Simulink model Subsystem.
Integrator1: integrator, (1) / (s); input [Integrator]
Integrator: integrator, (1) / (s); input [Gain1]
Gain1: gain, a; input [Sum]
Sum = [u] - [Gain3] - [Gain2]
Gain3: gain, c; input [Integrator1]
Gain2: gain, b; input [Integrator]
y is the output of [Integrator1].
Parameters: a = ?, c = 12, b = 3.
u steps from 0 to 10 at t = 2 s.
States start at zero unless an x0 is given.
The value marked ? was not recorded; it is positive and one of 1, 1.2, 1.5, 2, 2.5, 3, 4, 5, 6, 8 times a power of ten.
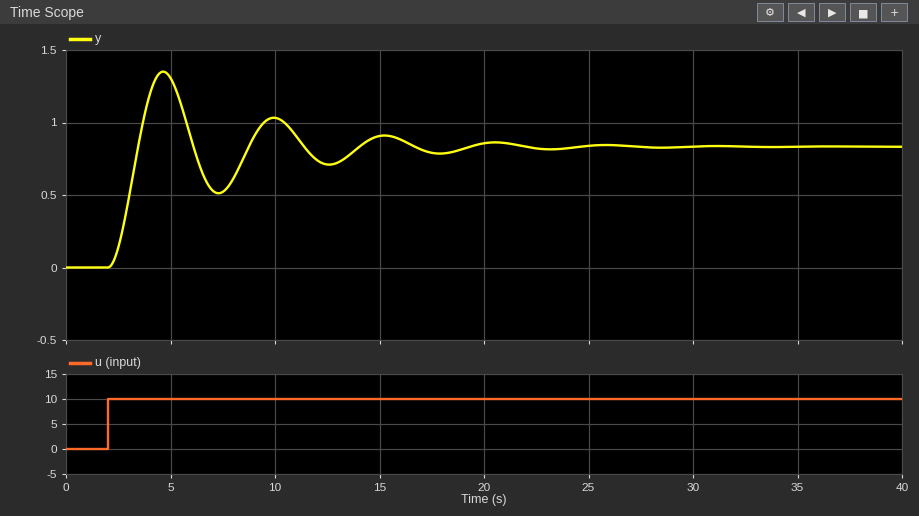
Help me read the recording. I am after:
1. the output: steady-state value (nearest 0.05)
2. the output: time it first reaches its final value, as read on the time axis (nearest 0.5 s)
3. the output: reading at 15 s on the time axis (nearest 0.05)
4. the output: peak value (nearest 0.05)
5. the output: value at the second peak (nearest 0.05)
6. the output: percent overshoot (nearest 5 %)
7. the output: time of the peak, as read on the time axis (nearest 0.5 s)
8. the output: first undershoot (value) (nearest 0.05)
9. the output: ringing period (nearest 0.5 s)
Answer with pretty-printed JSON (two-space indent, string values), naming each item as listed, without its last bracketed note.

{
  "the output: steady-state value": "0.85",
  "the output: time it first reaches its final value, as read on the time axis": "3.5 s",
  "the output: reading at 15 s on the time axis": "0.90",
  "the output: peak value": "1.35",
  "the output: value at the second peak": "1.05",
  "the output: percent overshoot": "60 %",
  "the output: time of the peak, as read on the time axis": "4.5 s",
  "the output: first undershoot (value)": "0.50",
  "the output: ringing period": "5.5 s"
}
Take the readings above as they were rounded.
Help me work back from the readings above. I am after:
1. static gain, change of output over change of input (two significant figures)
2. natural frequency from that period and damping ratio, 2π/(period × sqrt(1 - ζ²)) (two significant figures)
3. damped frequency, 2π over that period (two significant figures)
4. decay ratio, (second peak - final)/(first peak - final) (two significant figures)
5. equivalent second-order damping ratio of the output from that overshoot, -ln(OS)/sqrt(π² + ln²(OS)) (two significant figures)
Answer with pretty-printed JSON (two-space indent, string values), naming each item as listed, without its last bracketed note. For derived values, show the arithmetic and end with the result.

{
  "static gain, change of output over change of input": "(0.85 - 0) / (10 - 0) = 0.085",
  "natural frequency from that period and damping ratio, 2π/(period × sqrt(1 - ζ²))": "2π / (5.5 × sqrt(1 - 0.16²)) = 1.2 rad/s",
  "damped frequency, 2π over that period": "2π / 5.5 = 1.1 rad/s",
  "decay ratio, (second peak - final)/(first peak - final)": "(1.05 - 0.85) / (1.35 - 0.85) = 0.40",
  "equivalent second-order damping ratio of the output from that overshoot, -ln(OS)/sqrt(π² + ln²(OS))": "ln(0.6) = -0.511; 0.511 / sqrt(9.870 + 0.261) = 0.16"
}
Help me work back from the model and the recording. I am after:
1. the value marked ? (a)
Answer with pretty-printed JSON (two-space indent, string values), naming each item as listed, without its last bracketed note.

{
  "the value marked ?": "0.12"
}
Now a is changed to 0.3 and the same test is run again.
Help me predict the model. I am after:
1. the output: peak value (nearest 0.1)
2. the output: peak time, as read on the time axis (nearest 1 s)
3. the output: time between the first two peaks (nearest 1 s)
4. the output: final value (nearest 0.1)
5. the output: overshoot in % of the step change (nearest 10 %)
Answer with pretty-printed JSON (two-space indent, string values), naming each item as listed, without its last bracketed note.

{
  "the output: peak value": "1.2",
  "the output: peak time, as read on the time axis": "4 s",
  "the output: time between the first two peaks": "3 s",
  "the output: final value": "0.8",
  "the output: overshoot in % of the step change": "50 %"
}
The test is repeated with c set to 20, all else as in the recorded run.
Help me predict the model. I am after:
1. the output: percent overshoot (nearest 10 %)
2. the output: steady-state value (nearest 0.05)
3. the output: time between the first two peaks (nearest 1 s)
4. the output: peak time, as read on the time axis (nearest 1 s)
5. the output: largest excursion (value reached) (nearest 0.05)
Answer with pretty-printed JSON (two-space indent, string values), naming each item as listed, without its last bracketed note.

{
  "the output: percent overshoot": "70 %",
  "the output: steady-state value": "0.50",
  "the output: time between the first two peaks": "4 s",
  "the output: peak time, as read on the time axis": "4 s",
  "the output: largest excursion (value reached)": "0.85"
}
